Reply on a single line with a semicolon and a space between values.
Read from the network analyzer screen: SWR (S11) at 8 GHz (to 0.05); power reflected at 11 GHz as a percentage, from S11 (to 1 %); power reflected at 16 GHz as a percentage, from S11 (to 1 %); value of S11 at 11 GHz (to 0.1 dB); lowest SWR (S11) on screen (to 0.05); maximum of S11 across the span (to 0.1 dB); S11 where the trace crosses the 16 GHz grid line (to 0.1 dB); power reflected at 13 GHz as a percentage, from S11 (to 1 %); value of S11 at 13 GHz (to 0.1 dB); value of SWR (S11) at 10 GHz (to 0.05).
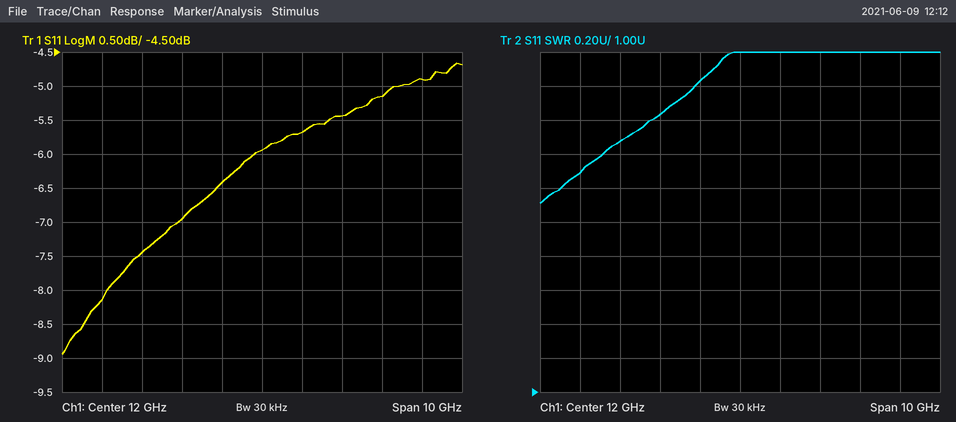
2.30; 23 %; 32 %; -6.4 dB; 2.10; -4.7 dB; -4.9 dB; 27 %; -5.7 dB; 2.65
